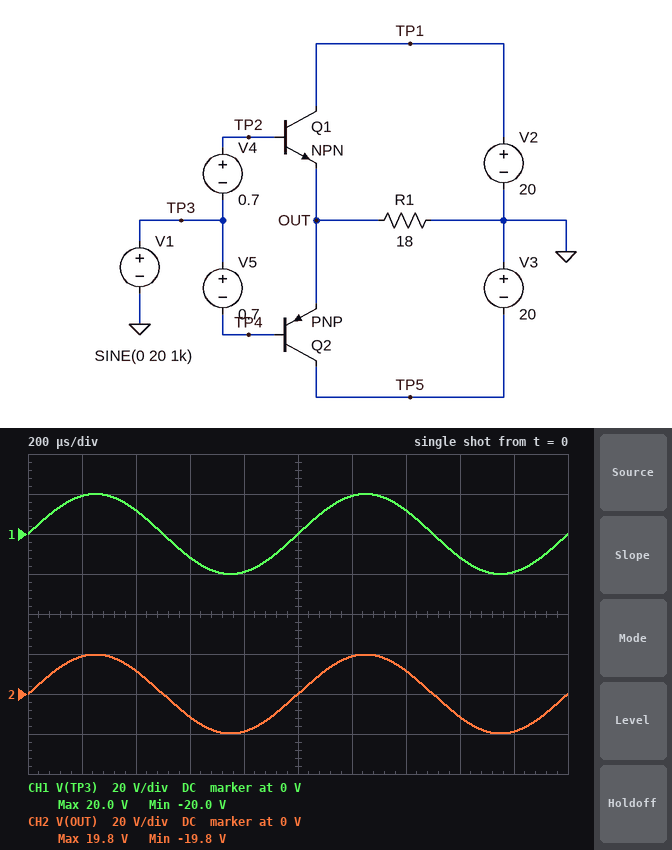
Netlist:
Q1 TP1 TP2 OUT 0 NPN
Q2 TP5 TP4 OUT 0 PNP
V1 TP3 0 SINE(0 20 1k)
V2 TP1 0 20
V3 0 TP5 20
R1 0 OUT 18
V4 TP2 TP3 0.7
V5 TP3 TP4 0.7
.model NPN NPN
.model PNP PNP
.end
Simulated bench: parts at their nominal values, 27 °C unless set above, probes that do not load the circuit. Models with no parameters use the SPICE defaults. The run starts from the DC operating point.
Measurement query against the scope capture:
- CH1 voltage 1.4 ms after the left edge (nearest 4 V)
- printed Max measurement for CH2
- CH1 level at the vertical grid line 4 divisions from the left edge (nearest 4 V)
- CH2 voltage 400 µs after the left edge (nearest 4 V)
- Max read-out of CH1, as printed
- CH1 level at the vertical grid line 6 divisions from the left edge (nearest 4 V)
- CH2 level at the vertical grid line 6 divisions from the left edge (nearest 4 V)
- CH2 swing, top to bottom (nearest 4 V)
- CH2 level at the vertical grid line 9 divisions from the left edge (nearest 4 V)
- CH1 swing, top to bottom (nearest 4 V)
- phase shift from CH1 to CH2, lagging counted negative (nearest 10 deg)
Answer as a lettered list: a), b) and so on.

a) 12 V
b) 19.8 V
c) -20 V
d) 12 V
e) 20.0 V
f) 20 V
g) 20 V
h) 40 V
i) -20 V
j) 40 V
k) 0 deg
